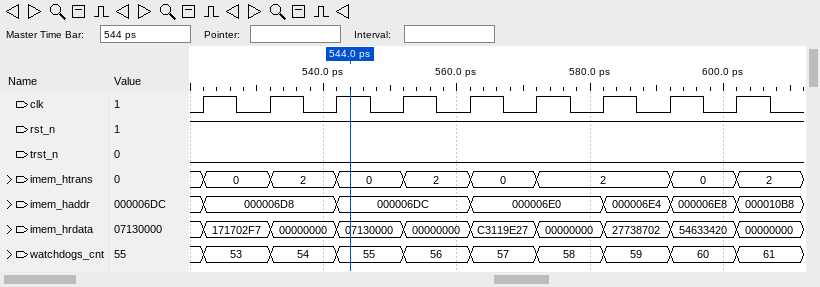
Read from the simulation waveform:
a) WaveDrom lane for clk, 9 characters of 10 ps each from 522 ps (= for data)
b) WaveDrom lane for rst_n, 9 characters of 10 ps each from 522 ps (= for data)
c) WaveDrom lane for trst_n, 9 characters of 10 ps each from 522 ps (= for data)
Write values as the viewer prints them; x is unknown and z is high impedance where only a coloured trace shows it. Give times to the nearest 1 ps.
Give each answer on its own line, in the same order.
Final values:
{name: 'clk', wave: 'p........'}
{name: 'rst_n', wave: '1........'}
{name: 'trst_n', wave: '0........'}
